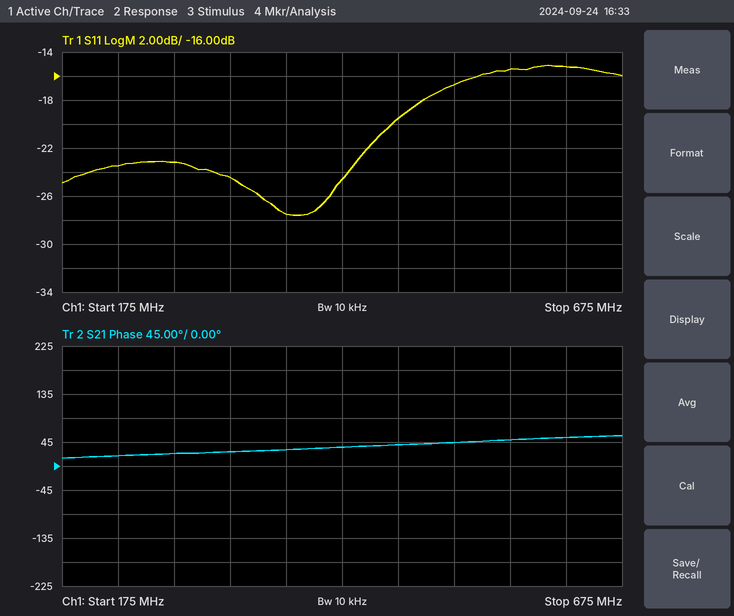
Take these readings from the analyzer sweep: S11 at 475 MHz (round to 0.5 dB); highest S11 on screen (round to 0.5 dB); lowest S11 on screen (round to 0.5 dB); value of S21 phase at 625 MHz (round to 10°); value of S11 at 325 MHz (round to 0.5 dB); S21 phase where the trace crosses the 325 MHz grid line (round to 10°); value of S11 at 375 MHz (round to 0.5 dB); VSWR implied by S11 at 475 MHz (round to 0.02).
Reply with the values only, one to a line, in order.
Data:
-19.5 dB
-15.0 dB
-27.5 dB
50°
-24.5 dB
30°
-27.5 dB
1.24
